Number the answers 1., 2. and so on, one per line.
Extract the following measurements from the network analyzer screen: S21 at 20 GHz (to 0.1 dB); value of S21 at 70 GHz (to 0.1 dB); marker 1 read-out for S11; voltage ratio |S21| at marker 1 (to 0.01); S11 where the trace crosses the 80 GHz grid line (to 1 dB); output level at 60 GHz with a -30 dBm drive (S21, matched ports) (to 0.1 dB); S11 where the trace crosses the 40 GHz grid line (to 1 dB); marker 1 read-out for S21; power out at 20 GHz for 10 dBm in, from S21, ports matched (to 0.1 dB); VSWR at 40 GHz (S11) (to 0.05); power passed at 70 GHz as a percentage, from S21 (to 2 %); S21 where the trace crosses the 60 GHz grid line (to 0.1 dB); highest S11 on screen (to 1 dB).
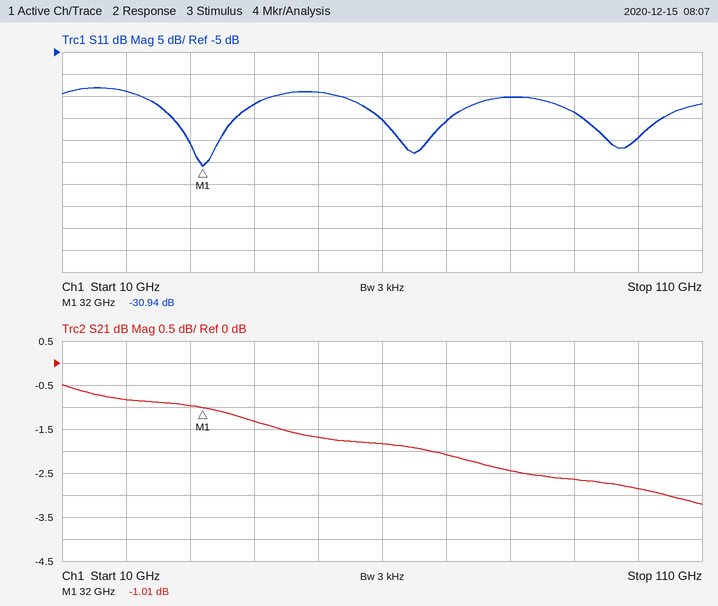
1. -0.8 dB
2. -2.1 dB
3. -30.94 dB
4. 0.89
5. -15 dB
6. -31.8 dBm
7. -17 dB
8. -1.01 dB
9. 9.2 dBm
10. 1.35
11. 62 %
12. -1.8 dB
13. -13 dB
